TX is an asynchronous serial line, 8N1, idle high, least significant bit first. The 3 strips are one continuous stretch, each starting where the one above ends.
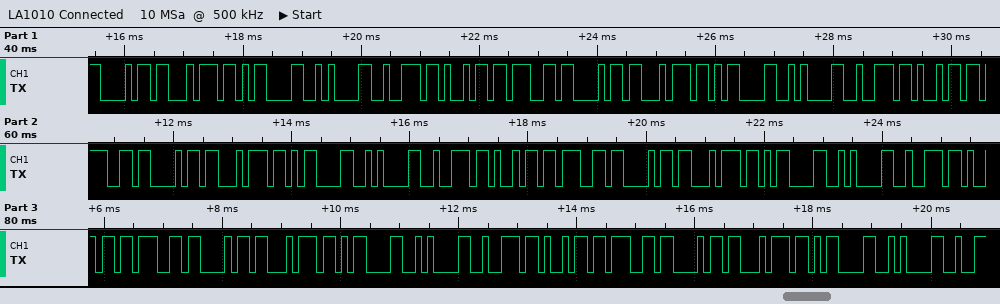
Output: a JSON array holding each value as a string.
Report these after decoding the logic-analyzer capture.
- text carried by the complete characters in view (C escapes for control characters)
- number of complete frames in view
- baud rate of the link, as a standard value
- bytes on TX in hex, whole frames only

["\"ht\\r\\nright\\r\\nright\\r\\nright\\r\\nright\\r\\nright\\r\\n\"", "39", "9600 baud", "68 74 0D 0A 72 69 67 68 74 0D 0A 72 69 67 68 74 0D 0A 72 69 67 68 74 0D 0A 72 69 67 68 74 0D 0A 72 69 67 68 74 0D 0A"]
